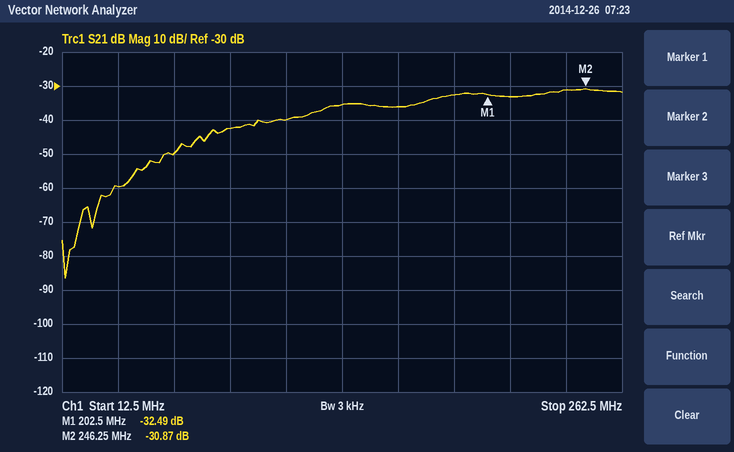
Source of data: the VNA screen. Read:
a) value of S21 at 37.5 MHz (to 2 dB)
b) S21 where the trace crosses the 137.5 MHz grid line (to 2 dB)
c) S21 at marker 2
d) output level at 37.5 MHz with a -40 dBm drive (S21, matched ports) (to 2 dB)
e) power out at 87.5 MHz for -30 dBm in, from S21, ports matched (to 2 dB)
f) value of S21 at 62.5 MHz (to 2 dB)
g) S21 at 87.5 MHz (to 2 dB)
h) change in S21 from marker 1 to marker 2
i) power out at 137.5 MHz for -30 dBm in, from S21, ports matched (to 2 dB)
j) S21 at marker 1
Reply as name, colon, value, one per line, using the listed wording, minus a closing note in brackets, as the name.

value of S21 at 37.5 MHz: -60 dB
S21 where the trace crosses the 137.5 MHz grid line: -36 dB
S21 at marker 2: -30.87 dB
output level at 37.5 MHz with a -40 dBm drive (S21, matched ports): -100 dBm
power out at 87.5 MHz for -30 dBm in, from S21, ports matched: -72 dBm
value of S21 at 62.5 MHz: -50 dB
S21 at 87.5 MHz: -42 dB
change in S21 from marker 1 to marker 2: 1.62 dB
power out at 137.5 MHz for -30 dBm in, from S21, ports matched: -66 dBm
S21 at marker 1: -32.49 dB
